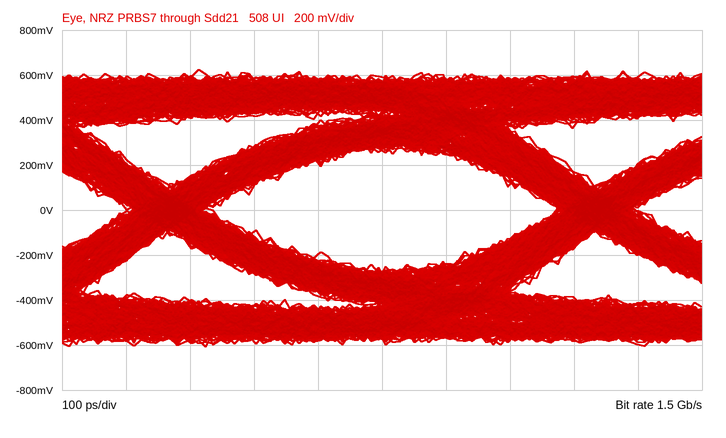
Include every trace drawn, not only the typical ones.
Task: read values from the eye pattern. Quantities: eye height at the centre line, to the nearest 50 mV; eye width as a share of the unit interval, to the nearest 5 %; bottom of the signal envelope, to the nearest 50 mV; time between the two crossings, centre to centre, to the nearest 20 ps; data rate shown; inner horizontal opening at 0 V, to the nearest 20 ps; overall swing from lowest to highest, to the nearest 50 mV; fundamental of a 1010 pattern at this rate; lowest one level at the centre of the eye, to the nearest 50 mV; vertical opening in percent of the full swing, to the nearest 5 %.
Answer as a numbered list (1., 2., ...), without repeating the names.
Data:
1. 550 mV
2. 80 %
3. -600 mV
4. 660 ps
5. 1.5 Gb/s
6. 540 ps
7. 1.25 V
8. 750 MHz
9. 250 mV
10. 45 %
